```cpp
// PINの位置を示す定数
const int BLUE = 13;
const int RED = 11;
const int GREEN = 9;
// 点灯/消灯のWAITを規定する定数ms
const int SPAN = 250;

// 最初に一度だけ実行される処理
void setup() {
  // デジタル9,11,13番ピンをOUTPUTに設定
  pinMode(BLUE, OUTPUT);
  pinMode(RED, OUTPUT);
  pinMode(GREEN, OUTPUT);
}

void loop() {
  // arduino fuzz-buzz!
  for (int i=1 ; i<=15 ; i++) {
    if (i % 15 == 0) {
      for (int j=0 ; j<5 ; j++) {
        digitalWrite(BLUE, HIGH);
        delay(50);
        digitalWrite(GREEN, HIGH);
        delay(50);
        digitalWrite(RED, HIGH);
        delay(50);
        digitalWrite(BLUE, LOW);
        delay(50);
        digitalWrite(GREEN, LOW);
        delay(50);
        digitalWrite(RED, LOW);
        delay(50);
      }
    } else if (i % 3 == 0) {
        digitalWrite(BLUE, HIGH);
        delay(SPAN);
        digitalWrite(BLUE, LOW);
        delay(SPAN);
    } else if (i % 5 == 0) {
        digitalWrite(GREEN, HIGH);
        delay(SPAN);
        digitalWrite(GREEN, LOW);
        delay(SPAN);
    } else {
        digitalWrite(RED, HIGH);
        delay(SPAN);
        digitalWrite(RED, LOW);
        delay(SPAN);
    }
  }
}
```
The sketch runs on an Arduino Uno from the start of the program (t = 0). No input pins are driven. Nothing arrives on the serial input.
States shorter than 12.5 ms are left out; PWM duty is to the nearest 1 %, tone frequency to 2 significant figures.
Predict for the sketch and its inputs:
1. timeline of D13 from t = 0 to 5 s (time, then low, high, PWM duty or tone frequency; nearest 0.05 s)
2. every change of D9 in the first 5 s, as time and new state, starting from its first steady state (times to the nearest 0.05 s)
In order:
0 s low; 1 s high; 1.25 s low; 2.5 s high; 2.75 s low; 4 s high; 4.25 s low
0 s low; 2 s high; 2.25 s low; 4.5 s high; 4.75 s low
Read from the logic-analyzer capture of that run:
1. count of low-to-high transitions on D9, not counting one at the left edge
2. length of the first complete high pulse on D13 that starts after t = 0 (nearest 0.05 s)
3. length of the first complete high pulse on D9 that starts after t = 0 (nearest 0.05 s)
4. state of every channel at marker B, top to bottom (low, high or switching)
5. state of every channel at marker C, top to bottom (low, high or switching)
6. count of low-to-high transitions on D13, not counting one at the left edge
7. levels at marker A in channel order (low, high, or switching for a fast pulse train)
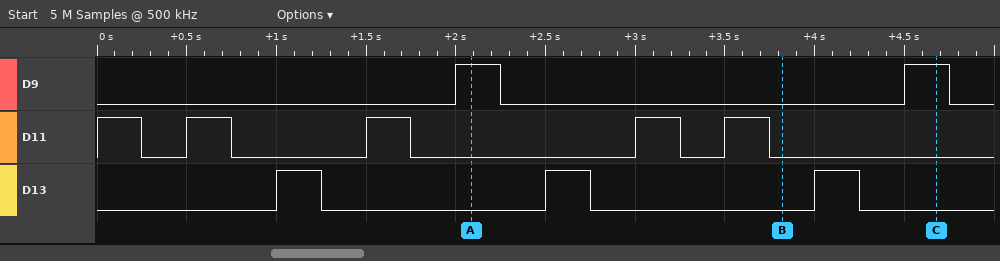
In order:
2
0.25 s
0.25 s
D9 low, D11 low, D13 low
D9 high, D11 low, D13 low
3
D9 high, D11 low, D13 low
